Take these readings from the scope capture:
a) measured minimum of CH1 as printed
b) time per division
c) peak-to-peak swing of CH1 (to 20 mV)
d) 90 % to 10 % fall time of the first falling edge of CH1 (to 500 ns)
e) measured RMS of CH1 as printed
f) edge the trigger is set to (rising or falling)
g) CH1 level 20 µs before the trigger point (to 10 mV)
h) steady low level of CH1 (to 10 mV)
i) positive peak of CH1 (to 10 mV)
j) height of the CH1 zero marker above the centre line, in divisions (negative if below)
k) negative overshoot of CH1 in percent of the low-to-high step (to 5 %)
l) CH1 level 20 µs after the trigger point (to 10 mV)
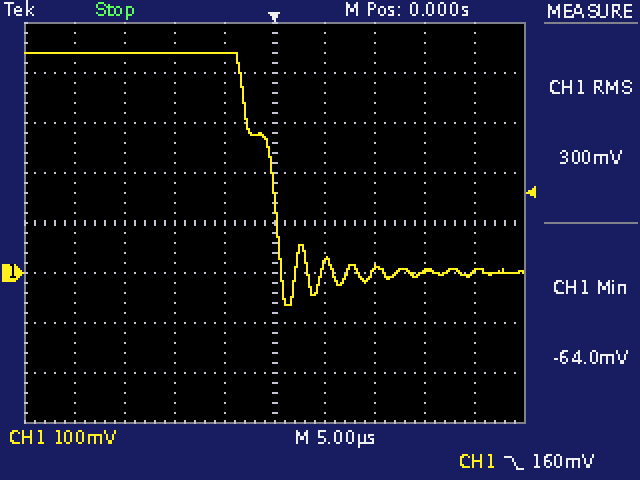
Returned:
-64.0 mV
5 µs
500 mV
4.0 µs
300 mV
falling
440 mV
0 mV
440 mV
-1.0 div
15 %
0 mV
